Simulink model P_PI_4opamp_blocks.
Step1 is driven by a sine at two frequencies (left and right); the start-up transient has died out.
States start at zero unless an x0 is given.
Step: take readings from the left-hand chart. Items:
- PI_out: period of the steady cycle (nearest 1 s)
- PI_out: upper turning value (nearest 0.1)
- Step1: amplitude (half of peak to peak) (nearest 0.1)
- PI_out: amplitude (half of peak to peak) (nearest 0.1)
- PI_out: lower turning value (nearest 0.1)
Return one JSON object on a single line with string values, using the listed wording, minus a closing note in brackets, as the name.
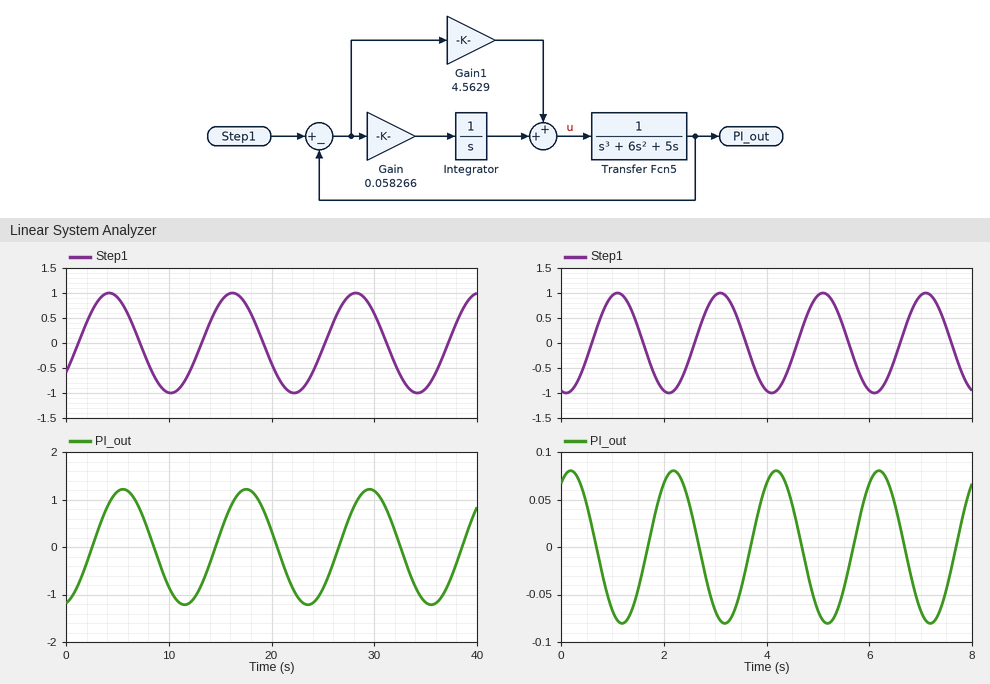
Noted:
{"PI_out: period of the steady cycle": "12 s", "PI_out: upper turning value": "1.2", "Step1: amplitude (half of peak to peak)": "1.0", "PI_out: amplitude (half of peak to peak)": "1.2", "PI_out: lower turning value": "-1.2"}
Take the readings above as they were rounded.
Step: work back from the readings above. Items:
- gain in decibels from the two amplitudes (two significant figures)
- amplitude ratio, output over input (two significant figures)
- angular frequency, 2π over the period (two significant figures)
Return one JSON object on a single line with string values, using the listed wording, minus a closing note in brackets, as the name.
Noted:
{"gain in decibels from the two amplitudes": "1.6 dB", "amplitude ratio, output over input": "1.2", "angular frequency, 2π over the period": "0.52 rad/s"}
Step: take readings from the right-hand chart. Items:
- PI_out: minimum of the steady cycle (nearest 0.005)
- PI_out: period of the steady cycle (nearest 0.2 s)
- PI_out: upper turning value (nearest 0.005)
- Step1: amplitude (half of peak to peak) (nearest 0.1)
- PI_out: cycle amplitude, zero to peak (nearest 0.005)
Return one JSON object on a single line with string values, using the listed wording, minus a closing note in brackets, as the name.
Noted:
{"PI_out: minimum of the steady cycle": "-0.080", "PI_out: period of the steady cycle": "2.0 s", "PI_out: upper turning value": "0.080", "Step1: amplitude (half of peak to peak)": "1.0", "PI_out: cycle amplitude, zero to peak": "0.080"}
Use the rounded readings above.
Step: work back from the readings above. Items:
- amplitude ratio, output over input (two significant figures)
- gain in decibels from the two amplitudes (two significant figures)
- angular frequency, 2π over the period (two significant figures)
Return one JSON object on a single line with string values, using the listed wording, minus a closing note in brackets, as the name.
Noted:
{"amplitude ratio, output over input": "0.080", "gain in decibels from the two amplitudes": "-22 dB", "angular frequency, 2π over the period": "3.1 rad/s"}
